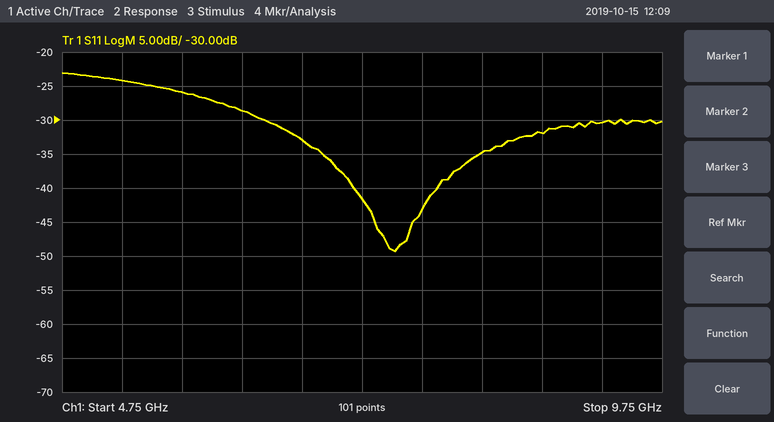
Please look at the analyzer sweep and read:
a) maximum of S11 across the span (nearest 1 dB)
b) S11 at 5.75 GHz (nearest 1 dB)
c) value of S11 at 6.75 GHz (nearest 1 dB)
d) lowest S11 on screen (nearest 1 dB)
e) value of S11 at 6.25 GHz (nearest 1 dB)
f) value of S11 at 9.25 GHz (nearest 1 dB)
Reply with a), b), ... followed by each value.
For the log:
a) -23 dB
b) -26 dB
c) -33 dB
d) -49 dB
e) -29 dB
f) -30 dB
